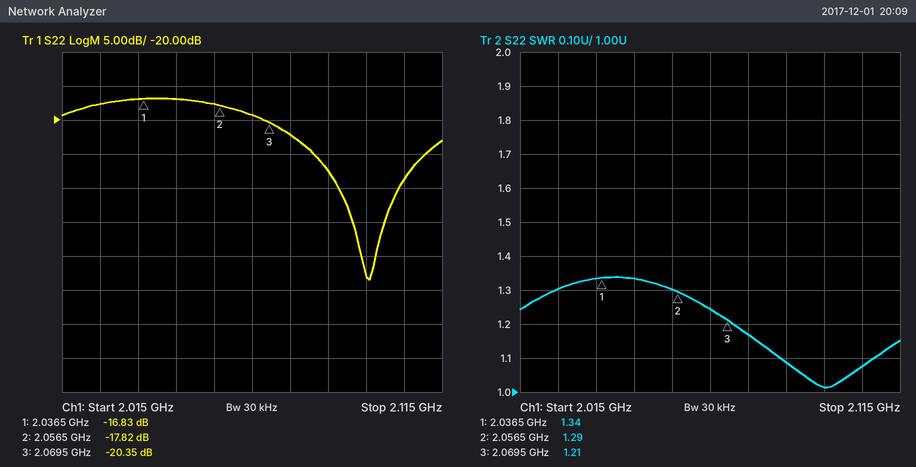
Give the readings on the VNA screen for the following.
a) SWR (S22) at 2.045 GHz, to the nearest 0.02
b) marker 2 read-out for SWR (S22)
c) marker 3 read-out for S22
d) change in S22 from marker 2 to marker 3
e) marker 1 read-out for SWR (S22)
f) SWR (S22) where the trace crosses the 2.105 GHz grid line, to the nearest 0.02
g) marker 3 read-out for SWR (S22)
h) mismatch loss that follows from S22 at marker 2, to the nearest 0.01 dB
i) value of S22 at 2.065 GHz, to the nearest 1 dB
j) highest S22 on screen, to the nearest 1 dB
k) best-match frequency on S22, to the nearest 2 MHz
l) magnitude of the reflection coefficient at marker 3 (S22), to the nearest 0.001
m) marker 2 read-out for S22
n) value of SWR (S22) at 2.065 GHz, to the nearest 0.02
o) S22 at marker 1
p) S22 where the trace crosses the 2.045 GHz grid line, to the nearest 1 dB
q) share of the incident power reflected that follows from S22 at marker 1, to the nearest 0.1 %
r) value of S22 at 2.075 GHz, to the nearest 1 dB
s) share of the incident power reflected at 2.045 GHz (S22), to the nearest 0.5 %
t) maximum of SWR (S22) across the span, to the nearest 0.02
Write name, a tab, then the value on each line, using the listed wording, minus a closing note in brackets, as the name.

SWR (S22) at 2.045 GHz, to the nearest 0.02	1.34
marker 2 read-out for SWR	1.29
marker 3 read-out for S22	-20.35 dB
change in S22 from marker 2 to marker 3	-2.53 dB
marker 1 read-out for SWR	1.34
SWR (S22) where the trace crosses the 2.105 GHz grid line, to the nearest 0.02	1.08
marker 3 read-out for SWR	1.21
mismatch loss that follows from S22 at marker 2, to the nearest 0.01 dB	0.07 dB
value of S22 at 2.065 GHz, to the nearest 1 dB	-19 dB
highest S22 on screen, to the nearest 1 dB	-17 dB
best-match frequency on S22, to the nearest 2 MHz	2.096 GHz
magnitude of the reflection coefficient at marker 3 (S22), to the nearest 0.001	0.096
marker 2 read-out for S22	-17.82 dB
value of SWR (S22) at 2.065 GHz, to the nearest 0.02	1.24
S22 at marker 1	-16.83 dB
S22 where the trace crosses the 2.045 GHz grid line, to the nearest 1 dB	-17 dB
share of the incident power reflected that follows from S22 at marker 1, to the nearest 0.1 %	2.1 %
value of S22 at 2.075 GHz, to the nearest 1 dB	-22 dB
share of the incident power reflected at 2.045 GHz (S22), to the nearest 0.5 %	2.0 %
maximum of SWR (S22) across the span, to the nearest 0.02	1.34
